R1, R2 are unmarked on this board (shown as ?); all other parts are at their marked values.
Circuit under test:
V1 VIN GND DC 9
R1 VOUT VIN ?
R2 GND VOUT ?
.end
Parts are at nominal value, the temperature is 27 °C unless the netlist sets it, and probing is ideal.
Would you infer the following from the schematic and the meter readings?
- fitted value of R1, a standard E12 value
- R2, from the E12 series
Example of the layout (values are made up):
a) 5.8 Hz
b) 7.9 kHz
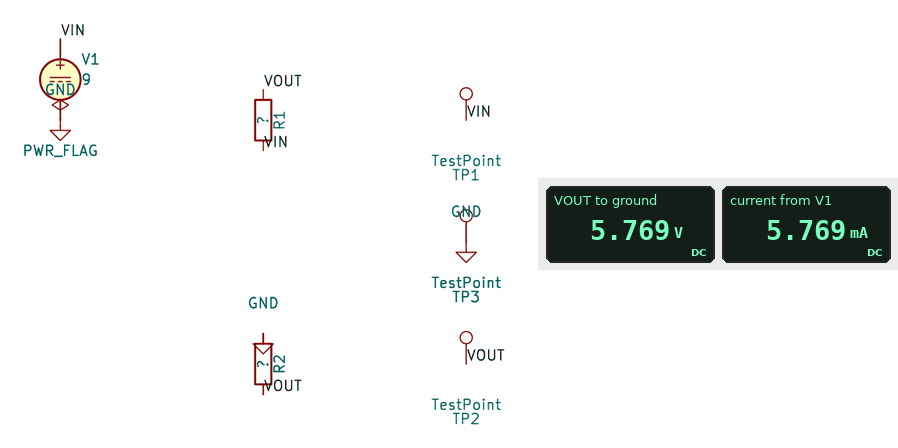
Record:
a) 560 Ω
b) 1 kΩ
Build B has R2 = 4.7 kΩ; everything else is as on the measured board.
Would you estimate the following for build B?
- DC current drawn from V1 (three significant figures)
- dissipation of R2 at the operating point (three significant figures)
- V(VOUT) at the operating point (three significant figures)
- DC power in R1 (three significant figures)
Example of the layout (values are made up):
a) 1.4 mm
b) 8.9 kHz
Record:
a) 1.71 mA
b) 13.8 mW
c) 8.04 V
d) 1.64 mW
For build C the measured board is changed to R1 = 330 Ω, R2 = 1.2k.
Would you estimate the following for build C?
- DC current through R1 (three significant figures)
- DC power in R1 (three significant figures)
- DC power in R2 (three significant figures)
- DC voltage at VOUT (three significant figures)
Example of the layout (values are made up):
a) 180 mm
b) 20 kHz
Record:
a) 5.88 mA
b) 11.4 mW
c) 41.5 mW
d) 7.06 V
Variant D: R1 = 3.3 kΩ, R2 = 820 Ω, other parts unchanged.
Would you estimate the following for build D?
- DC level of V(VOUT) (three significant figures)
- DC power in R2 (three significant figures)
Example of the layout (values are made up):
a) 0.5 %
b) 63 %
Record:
a) 1.79 V
b) 3.91 mW
